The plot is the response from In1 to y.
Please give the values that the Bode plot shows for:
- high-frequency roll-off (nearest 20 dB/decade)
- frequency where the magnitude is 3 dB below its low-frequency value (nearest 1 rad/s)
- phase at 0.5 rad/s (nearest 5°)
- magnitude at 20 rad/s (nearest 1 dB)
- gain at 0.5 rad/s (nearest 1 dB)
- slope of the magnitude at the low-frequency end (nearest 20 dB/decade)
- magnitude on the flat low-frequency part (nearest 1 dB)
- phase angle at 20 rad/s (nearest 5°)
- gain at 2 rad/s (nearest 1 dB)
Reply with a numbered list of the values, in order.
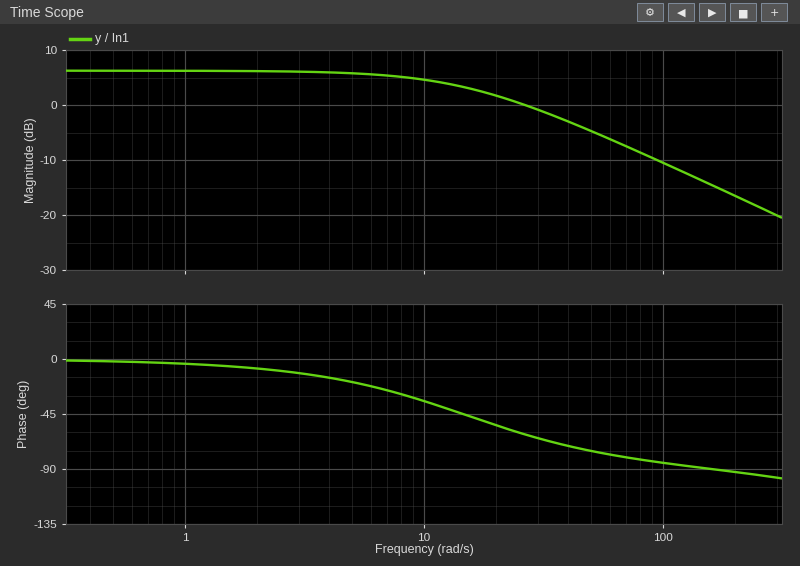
1. -20 dB/decade
2. 15 rad/s
3. 0°
4. 2 dB
5. 6 dB
6. 0 dB/decade
7. 6 dB
8. -55°
9. 6 dB
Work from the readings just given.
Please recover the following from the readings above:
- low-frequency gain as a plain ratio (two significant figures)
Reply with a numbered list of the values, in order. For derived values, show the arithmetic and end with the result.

1. 10^(6 / 20) = 2.0
